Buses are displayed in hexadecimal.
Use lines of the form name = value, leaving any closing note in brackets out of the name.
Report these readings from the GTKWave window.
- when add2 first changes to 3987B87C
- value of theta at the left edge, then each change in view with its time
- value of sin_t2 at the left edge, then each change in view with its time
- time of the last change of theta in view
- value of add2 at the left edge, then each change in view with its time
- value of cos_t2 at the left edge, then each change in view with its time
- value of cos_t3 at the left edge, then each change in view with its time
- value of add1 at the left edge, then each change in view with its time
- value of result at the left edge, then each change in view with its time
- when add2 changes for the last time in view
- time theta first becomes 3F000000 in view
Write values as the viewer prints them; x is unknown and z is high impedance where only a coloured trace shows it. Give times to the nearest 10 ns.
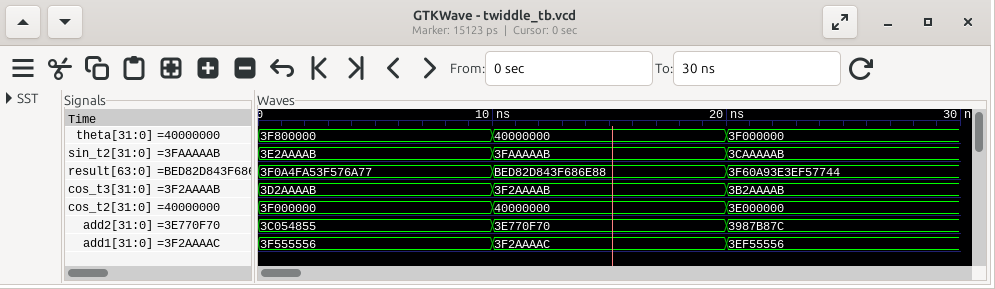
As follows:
when add2 first changes to 3987B87C = 20 ns
value of theta at the left edge, then each change in view with its time = 3F800000, 40000000 at 10 ns, 3F000000 at 20 ns
value of sin_t2 at the left edge, then each change in view with its time = 3E2AAAAB, 3FAAAAAB at 10 ns, 3CAAAAAB at 20 ns
time of the last change of theta in view = 20 ns
value of add2 at the left edge, then each change in view with its time = 3C054855, 3E770F70 at 10 ns, 3987B87C at 20 ns
value of cos_t2 at the left edge, then each change in view with its time = 3F000000, 40000000 at 10 ns, 3E000000 at 20 ns
value of cos_t3 at the left edge, then each change in view with its time = 3D2AAAAB, 3F2AAAAB at 10 ns, 3B2AAAAB at 20 ns
value of add1 at the left edge, then each change in view with its time = 3F555556, 3F2AAAAC at 10 ns, 3EF55556 at 20 ns
value of result at the left edge, then each change in view with its time = 3F0A4FA53F576A77, BED82D843F686E88 at 10 ns, 3F60A93E3EF57744 at 20 ns
when add2 changes for the last time in view = 20 ns
time theta first becomes 3F000000 in view = 20 ns
